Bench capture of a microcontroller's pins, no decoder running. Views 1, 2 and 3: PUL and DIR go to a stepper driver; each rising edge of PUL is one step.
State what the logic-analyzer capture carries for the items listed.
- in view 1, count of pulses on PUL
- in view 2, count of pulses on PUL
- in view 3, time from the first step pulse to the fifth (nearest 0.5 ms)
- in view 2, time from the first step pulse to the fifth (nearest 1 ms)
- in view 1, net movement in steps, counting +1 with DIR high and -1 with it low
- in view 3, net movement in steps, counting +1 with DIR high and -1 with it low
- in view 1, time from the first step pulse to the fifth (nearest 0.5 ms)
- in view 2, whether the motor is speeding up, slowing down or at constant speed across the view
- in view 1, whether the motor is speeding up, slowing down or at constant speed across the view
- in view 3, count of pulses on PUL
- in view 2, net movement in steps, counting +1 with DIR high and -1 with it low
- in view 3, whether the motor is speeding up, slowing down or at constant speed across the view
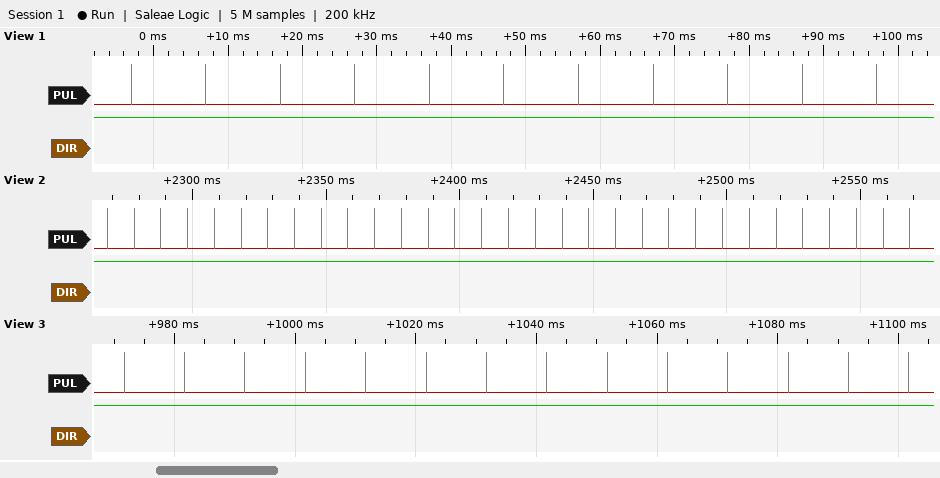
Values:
11
31
40.0 ms
40 ms
+11
+14
40.0 ms
constant speed
constant speed
14
+31
constant speed
